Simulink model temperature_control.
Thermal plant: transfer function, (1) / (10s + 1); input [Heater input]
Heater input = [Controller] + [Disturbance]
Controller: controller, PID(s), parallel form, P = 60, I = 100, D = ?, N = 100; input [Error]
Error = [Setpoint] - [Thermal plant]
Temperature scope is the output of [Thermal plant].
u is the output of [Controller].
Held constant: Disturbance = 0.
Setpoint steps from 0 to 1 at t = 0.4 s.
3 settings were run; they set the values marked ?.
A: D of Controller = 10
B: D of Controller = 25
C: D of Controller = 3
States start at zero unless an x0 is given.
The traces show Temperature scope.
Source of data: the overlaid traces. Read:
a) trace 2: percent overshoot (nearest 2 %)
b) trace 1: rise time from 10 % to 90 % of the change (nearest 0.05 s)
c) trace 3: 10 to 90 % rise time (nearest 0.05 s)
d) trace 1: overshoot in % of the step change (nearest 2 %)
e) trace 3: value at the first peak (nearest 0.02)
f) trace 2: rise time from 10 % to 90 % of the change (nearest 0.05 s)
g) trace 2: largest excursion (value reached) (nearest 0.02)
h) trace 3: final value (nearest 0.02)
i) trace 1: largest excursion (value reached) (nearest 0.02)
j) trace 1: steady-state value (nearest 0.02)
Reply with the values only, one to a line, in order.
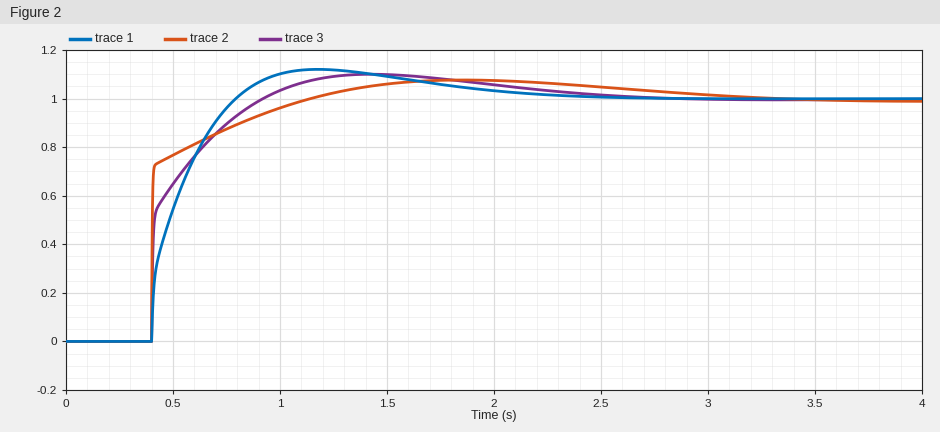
8 %
0.30 s
0.35 s
12 %
1.10
0.40 s
1.08
1.00
1.12
1.00
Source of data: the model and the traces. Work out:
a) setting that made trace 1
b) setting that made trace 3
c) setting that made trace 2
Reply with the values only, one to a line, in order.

C
A
B
